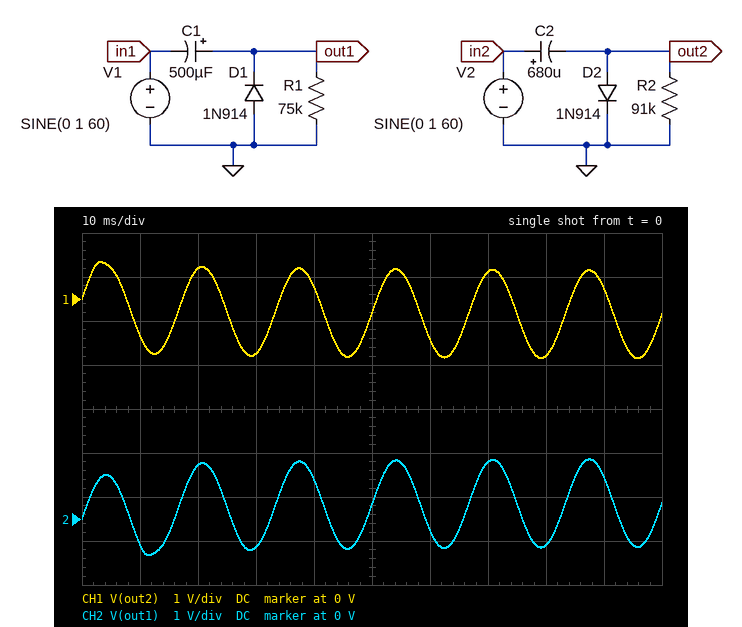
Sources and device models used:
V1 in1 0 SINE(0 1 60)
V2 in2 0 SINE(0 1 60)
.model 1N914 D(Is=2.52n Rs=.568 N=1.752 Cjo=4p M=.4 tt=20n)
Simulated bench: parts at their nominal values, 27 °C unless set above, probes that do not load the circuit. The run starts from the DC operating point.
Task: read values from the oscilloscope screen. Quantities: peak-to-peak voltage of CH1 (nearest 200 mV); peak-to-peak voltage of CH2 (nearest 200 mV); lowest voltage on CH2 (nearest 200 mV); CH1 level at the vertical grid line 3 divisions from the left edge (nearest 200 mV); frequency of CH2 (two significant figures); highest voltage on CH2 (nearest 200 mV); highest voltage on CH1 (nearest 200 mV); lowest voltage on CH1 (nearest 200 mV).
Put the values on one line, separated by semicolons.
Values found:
2.2 V; 2.2 V; -800 mV; -1.2 V; 60 Hz; 1.4 V; 800 mV; -1.4 V
